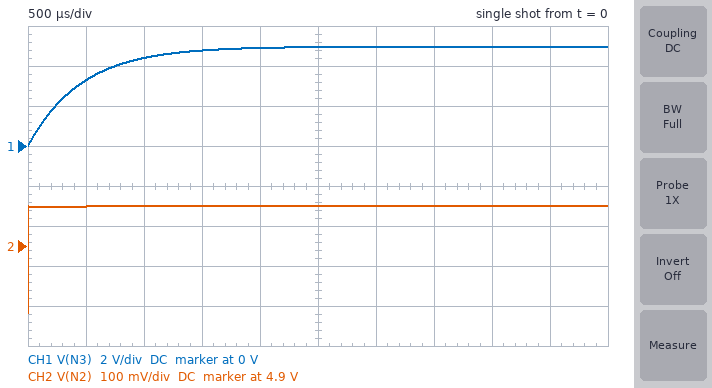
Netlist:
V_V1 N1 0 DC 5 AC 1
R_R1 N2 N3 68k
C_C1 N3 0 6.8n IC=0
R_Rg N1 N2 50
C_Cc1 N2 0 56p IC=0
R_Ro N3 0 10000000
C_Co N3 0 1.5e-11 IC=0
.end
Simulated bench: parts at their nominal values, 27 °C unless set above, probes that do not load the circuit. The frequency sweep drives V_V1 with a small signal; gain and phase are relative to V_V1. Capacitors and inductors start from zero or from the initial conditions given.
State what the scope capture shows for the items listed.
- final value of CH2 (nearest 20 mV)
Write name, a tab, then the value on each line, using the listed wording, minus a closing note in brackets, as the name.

final value of CH2	5.00 V
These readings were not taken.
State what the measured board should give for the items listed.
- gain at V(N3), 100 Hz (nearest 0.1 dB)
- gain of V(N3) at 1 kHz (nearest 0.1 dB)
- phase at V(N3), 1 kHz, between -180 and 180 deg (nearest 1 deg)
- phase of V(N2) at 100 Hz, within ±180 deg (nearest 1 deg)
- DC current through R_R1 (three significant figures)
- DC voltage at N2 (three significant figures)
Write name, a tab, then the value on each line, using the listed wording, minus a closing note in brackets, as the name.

gain at V(N3), 100 Hz	-0.4 dB
gain of V(N3) at 1 kHz	-9.8 dB
phase at V(N3), 1 kHz, between -180 and 180 deg	-71 deg
phase of V(N2) at 100 Hz, within ±180 deg	0 deg
DC current through R_R1	497 nA
DC voltage at N2	5.00 V
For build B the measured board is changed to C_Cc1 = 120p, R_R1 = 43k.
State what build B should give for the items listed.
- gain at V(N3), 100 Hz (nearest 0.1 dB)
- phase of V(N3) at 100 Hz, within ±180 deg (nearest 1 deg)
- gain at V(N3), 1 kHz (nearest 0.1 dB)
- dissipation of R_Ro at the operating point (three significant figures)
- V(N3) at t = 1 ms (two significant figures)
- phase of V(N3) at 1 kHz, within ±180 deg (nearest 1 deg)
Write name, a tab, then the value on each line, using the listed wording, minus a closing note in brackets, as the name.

gain at V(N3), 100 Hz	-0.2 dB
phase of V(N3) at 100 Hz, within ±180 deg	-10 deg
gain at V(N3), 1 kHz	-6.4 dB
dissipation of R_Ro at the operating point	2.48 µW
V(N3) at t = 1 ms	4.8 V
phase of V(N3) at 1 kHz, within ±180 deg	-61 deg
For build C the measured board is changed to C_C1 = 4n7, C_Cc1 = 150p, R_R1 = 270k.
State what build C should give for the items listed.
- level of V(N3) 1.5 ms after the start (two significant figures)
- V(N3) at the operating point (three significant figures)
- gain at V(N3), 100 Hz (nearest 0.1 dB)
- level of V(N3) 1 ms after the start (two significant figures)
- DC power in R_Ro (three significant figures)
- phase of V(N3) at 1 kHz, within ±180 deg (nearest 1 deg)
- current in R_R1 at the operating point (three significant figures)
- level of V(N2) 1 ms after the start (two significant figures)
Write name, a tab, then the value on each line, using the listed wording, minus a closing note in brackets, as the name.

level of V(N3) 1.5 ms after the start	3.4 V
V(N3) at the operating point	4.87 V
gain at V(N3), 100 Hz	-2.3 dB
level of V(N3) 1 ms after the start	2.7 V
DC power in R_Ro	2.37 µW
phase of V(N3) at 1 kHz, within ±180 deg	-83 deg
current in R_R1 at the operating point	487 nA
level of V(N2) 1 ms after the start	5.0 V
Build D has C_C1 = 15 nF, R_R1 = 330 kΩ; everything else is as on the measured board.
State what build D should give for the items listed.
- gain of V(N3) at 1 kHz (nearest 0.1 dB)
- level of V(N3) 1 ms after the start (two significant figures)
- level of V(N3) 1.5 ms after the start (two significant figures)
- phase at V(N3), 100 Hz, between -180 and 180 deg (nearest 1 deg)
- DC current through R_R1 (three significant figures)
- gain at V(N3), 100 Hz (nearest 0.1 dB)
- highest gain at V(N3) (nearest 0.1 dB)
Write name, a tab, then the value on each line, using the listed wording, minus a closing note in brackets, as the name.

gain of V(N3) at 1 kHz	-29.9 dB
level of V(N3) 1 ms after the start	910 mV
level of V(N3) 1.5 ms after the start	1.3 V
phase at V(N3), 100 Hz, between -180 and 180 deg	-72 deg
DC current through R_R1	484 nA
gain at V(N3), 100 Hz	-10.3 dB
highest gain at V(N3)	-0.3 dB
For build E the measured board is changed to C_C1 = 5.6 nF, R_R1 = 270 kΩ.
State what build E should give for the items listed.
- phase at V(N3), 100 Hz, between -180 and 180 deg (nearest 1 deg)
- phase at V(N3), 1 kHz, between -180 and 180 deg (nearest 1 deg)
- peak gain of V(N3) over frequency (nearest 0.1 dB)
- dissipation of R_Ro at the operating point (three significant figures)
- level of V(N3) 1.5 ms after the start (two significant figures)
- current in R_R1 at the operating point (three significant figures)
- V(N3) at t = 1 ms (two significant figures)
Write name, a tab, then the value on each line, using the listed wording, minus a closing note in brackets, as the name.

phase at V(N3), 100 Hz, between -180 and 180 deg	-43 deg
phase at V(N3), 1 kHz, between -180 and 180 deg	-84 deg
peak gain of V(N3) over frequency	-0.2 dB
dissipation of R_Ro at the operating point	2.37 µW
level of V(N3) 1.5 ms after the start	3.1 V
current in R_R1 at the operating point	487 nA
V(N3) at t = 1 ms	2.4 V
